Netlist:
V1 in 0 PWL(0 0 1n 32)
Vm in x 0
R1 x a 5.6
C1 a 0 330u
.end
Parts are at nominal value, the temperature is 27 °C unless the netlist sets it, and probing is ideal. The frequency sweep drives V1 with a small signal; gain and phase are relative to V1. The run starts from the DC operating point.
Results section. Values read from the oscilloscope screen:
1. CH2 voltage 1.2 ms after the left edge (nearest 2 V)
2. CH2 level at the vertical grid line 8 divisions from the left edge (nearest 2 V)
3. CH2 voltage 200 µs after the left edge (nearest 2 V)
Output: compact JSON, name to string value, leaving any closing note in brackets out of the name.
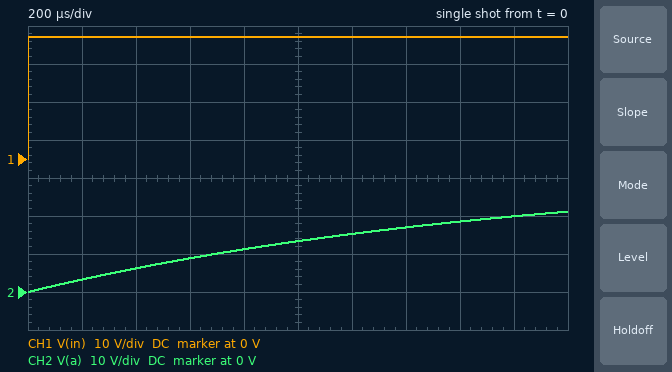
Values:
{"CH2 voltage 1.2 ms after the left edge": "16 V", "CH2 level at the vertical grid line 8 divisions from the left edge": "18 V", "CH2 voltage 200 µs after the left edge": "4 V"}
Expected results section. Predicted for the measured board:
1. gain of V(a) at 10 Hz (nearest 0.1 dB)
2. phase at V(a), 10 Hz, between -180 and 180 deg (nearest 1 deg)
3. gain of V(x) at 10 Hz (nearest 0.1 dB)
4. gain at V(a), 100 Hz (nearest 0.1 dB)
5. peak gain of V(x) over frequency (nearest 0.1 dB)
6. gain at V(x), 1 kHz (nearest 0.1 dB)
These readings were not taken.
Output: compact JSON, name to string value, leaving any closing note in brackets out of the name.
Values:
{"gain of V(a) at 10 Hz": "-0.1 dB", "phase at V(a), 10 Hz, between -180 and 180 deg": "-7 deg", "gain of V(x) at 10 Hz": "0 dB", "gain at V(a), 100 Hz": "-3.7 dB", "peak gain of V(x) over frequency": "0 dB", "gain at V(x), 1 kHz": "0 dB"}
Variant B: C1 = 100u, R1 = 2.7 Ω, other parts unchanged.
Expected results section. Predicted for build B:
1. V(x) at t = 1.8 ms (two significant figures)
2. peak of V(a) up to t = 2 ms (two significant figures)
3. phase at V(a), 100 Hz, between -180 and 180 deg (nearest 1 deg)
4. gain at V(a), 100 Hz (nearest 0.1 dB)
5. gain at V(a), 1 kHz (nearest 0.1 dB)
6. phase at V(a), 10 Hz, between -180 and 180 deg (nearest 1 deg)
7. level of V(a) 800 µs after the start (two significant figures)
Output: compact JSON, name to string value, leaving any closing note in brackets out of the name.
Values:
{"V(x) at t = 1.8 ms": "32 V", "peak of V(a) up to t = 2 ms": "32 V", "phase at V(a), 100 Hz, between -180 and 180 deg": "-10 deg", "gain at V(a), 100 Hz": "-0.1 dB", "gain at V(a), 1 kHz": "-5.9 dB", "phase at V(a), 10 Hz, between -180 and 180 deg": "-1 deg", "level of V(a) 800 µs after the start": "30 V"}
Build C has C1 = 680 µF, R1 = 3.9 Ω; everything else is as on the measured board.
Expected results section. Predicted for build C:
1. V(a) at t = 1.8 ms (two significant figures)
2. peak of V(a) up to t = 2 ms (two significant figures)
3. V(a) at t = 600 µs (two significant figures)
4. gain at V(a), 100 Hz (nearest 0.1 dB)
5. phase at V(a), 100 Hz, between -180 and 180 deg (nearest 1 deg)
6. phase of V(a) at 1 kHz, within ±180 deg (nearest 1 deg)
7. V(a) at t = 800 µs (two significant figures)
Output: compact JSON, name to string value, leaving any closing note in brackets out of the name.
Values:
{"V(a) at t = 1.8 ms": "16 V", "peak of V(a) up to t = 2 ms": "17 V", "V(a) at t = 600 µs": "6.5 V", "gain at V(a), 100 Hz": "-5.8 dB", "phase at V(a), 100 Hz, between -180 and 180 deg": "-59 deg", "phase of V(a) at 1 kHz, within ±180 deg": "-87 deg", "V(a) at t = 800 µs": "8.3 V"}
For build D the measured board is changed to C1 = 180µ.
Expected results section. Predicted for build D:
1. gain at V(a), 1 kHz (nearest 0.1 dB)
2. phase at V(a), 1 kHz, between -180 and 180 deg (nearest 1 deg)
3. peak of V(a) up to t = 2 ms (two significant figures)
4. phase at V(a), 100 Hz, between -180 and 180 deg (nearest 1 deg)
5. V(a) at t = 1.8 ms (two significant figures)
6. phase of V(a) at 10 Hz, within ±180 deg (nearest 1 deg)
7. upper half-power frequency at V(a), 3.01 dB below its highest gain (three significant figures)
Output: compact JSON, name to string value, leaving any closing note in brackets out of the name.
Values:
{"gain at V(a), 1 kHz": "-16.1 dB", "phase at V(a), 1 kHz, between -180 and 180 deg": "-81 deg", "peak of V(a) up to t = 2 ms": "28 V", "phase at V(a), 100 Hz, between -180 and 180 deg": "-32 deg", "V(a) at t = 1.8 ms": "27 V", "phase of V(a) at 10 Hz, within ±180 deg": "-4 deg", "upper half-power frequency at V(a), 3.01 dB below its highest gain": "158 Hz"}
